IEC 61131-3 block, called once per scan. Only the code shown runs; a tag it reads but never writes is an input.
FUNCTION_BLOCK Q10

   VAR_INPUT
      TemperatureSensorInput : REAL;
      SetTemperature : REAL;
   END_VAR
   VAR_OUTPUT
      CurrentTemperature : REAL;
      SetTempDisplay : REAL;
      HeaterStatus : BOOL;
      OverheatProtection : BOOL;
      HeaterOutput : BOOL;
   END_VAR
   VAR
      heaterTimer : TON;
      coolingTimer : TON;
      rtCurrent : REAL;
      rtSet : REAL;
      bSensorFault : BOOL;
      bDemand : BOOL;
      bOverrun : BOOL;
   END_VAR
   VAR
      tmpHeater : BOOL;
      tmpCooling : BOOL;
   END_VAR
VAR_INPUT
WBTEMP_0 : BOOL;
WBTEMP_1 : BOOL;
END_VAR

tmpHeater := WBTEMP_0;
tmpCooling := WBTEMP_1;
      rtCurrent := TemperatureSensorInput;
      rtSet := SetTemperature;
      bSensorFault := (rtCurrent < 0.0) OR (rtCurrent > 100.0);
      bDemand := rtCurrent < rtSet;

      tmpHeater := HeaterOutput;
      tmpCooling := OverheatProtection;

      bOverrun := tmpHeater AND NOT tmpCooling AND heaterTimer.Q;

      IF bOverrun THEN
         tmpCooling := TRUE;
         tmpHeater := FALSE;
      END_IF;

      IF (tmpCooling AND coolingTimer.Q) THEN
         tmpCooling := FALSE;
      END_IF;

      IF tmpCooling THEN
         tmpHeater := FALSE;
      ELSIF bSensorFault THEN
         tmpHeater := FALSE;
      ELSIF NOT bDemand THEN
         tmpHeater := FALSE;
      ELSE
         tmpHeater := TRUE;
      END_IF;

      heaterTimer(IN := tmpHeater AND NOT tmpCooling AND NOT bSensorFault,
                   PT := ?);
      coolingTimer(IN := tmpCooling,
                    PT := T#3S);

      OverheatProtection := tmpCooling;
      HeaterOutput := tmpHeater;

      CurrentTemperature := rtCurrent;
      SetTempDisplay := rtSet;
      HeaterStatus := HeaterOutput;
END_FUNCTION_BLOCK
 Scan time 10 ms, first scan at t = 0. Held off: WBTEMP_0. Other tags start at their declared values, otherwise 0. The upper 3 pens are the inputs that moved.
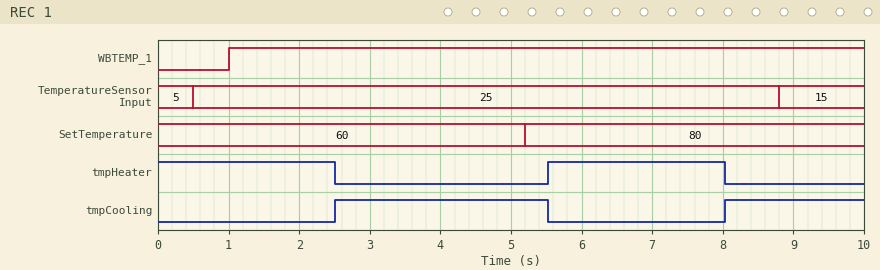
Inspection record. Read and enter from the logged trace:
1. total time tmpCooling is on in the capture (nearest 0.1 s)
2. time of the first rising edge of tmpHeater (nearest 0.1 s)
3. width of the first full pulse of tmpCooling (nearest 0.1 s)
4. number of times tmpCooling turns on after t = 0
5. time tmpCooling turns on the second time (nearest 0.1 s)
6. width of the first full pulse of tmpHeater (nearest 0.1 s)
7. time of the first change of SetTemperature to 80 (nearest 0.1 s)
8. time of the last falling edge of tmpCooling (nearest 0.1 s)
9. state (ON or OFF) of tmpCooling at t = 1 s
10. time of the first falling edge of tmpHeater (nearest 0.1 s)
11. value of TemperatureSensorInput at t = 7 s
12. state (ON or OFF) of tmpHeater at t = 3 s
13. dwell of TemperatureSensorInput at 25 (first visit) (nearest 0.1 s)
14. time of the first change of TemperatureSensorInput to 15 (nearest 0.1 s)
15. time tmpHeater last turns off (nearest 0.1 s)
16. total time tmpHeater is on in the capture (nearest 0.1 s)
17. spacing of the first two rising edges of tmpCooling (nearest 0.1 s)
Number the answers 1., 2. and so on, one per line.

1. 5.0 s
2. 5.5 s
3. 3.0 s
4. 2
5. 8.0 s
6. 2.5 s
7. 5.2 s
8. 5.5 s
9. OFF
10. 2.5 s
11. 25
12. OFF
13. 8.3 s
14. 8.8 s
15. 8.0 s
16. 5.0 s
17. 5.5 s
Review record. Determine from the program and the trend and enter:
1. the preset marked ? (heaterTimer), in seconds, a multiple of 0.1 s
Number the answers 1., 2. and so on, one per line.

1. 2.5 s
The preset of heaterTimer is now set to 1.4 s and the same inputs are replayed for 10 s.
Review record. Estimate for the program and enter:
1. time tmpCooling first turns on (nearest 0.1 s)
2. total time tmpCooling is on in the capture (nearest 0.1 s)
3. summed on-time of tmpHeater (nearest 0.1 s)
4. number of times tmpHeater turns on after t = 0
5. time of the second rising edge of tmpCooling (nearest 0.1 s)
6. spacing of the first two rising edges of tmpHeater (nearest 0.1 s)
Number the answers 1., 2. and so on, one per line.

1. 1.4 s
2. 6.0 s
3. 4.0 s
4. 2
5. 5.8 s
6. 4.4 s
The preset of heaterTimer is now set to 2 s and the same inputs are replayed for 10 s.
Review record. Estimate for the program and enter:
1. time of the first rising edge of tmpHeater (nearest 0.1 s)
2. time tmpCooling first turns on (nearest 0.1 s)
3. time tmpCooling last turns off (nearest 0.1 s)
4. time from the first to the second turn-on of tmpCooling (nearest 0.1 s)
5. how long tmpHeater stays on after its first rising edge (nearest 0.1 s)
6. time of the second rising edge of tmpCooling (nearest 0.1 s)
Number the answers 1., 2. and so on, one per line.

1. 5.0 s
2. 2.0 s
3. 5.0 s
4. 5.0 s
5. 2.0 s
6. 7.0 s
